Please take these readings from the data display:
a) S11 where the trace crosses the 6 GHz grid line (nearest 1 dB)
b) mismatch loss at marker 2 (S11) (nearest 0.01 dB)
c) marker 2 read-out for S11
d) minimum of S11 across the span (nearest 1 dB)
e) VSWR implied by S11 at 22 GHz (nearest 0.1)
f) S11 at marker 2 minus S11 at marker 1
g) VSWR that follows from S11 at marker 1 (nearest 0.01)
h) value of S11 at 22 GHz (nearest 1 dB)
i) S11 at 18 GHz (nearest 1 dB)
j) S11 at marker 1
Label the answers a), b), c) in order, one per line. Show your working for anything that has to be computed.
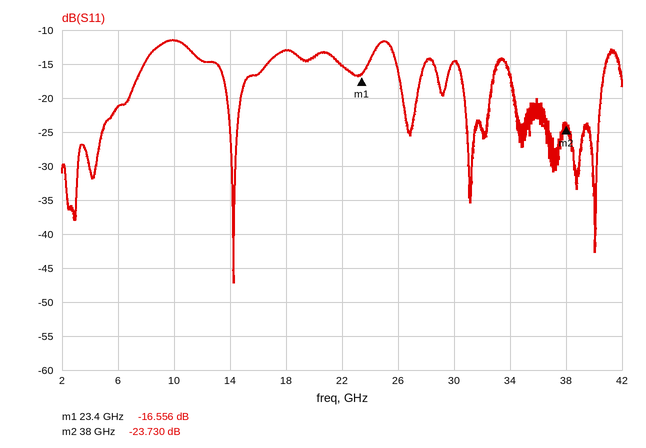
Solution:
a) -21 dB
b) −10 log10(1 − 10^(-23.73/10)) ≈ 0.02 dB
c) -23.730 dB
d) -47 dB
e) |Γ| = 10^(-15/20) = 0.1778; VSWR = (1 + 0.1778)/(1 − 0.1778) ≈ 1.4
f) -23.73 − (-16.556) = -7.174 dB
g) (1 + 0.1487)/(1 − 0.1487) ≈ 1.35
h) -15 dB
i) -13 dB
j) -16.556 dB
